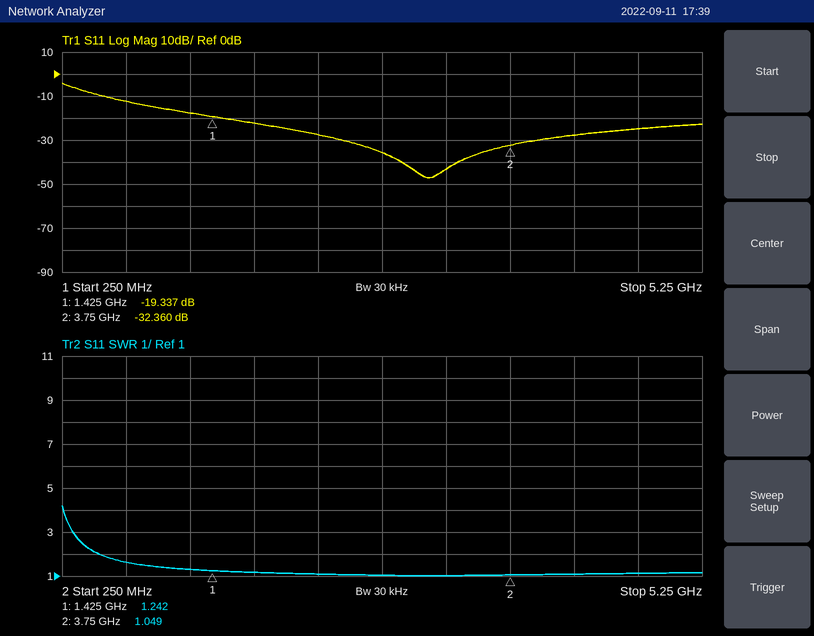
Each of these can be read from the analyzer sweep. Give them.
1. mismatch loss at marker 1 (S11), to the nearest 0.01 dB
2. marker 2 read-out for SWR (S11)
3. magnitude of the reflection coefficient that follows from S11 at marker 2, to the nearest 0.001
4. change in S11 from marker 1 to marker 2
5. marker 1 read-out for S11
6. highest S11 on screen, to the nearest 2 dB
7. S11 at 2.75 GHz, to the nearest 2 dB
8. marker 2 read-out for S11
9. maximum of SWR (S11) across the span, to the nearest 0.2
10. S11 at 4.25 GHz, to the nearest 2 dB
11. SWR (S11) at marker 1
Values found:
0.05 dB
1.049
0.024
-13.023 dB
-19.337 dB
-4 dB
-36 dB
-32.360 dB
4.2
-28 dB
1.242
